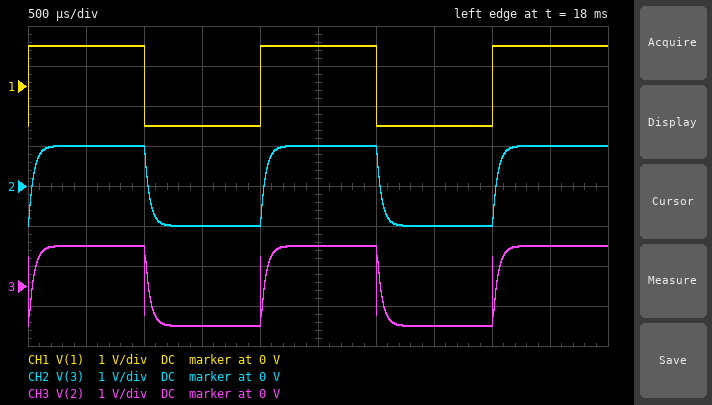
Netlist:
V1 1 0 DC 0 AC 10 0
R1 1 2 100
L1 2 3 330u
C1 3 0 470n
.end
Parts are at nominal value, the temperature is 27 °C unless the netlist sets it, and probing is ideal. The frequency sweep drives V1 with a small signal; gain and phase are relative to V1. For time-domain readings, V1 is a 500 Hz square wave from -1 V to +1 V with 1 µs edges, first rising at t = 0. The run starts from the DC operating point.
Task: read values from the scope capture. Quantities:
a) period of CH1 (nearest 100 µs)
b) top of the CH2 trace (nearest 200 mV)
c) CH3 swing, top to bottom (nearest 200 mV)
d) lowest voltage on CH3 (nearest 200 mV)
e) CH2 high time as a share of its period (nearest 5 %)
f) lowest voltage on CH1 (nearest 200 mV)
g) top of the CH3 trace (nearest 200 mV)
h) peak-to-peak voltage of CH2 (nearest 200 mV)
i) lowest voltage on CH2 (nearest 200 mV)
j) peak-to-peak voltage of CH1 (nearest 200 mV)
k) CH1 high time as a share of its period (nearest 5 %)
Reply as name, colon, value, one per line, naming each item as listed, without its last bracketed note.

period of CH1: 2.0 ms
top of the CH2 trace: 1.0 V
CH3 swing, top to bottom: 2.0 V
lowest voltage on CH3: -1.0 V
CH2 high time as a share of its period: 50 %
lowest voltage on CH1: -1.0 V
top of the CH3 trace: 1.0 V
peak-to-peak voltage of CH2: 2.0 V
lowest voltage on CH2: -1.0 V
peak-to-peak voltage of CH1: 2.0 V
CH1 high time as a share of its period: 50 %
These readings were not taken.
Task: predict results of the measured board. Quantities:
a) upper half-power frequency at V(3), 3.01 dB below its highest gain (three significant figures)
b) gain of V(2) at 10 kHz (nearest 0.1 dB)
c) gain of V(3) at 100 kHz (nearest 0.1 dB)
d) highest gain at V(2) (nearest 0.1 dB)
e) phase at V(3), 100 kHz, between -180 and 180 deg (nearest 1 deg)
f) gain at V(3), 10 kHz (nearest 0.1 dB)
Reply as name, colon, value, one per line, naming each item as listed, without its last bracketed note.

upper half-power frequency at V(3), 3.01 dB below its highest gain: 3.64 kHz
gain of V(2) at 10 kHz: -17.7 dB
gain of V(3) at 100 kHz: -36.5 dB
highest gain at V(2): 0 dB
phase at V(3), 100 kHz, between -180 and 180 deg: -154 deg
gain at V(3), 10 kHz: -9.5 dB
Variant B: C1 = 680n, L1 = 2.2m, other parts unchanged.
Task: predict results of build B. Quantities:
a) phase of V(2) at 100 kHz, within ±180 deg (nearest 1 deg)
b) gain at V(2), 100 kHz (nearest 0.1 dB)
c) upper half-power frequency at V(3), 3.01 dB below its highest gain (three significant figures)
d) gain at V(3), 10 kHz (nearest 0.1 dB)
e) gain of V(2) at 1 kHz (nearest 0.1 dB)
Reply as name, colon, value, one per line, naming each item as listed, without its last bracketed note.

phase of V(2) at 100 kHz, within ±180 deg: 4 deg
gain at V(2), 100 kHz: 0 dB
upper half-power frequency at V(3), 3.01 dB below its highest gain: 3.17 kHz
gain at V(3), 10 kHz: -16.3 dB
gain of V(2) at 1 kHz: -0.8 dB
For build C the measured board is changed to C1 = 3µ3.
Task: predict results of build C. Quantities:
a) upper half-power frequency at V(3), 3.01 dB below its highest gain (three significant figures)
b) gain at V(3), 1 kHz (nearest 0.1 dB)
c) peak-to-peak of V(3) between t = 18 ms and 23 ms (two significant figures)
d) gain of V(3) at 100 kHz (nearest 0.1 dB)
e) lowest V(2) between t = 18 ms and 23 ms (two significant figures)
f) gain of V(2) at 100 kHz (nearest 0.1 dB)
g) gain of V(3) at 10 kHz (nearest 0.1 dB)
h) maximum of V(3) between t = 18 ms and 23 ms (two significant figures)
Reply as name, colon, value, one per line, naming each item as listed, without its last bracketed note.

upper half-power frequency at V(3), 3.01 dB below its highest gain: 487 Hz
gain at V(3), 1 kHz: -7.2 dB
peak-to-peak of V(3) between t = 18 ms and 23 ms: 1.8 V
gain of V(3) at 100 kHz: -53.6 dB
lowest V(2) between t = 18 ms and 23 ms: -910 mV
gain of V(2) at 100 kHz: -0.9 dB
gain of V(3) at 10 kHz: -26.4 dB
maximum of V(3) between t = 18 ms and 23 ms: 910 mV
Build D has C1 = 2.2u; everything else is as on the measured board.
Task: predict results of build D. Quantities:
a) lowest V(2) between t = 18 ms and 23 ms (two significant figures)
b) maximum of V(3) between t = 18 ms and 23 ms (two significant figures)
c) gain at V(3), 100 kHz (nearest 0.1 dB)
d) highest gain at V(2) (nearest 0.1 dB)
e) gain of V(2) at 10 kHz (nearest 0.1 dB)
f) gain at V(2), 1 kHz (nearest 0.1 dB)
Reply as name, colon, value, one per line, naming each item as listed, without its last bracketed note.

lowest V(2) between t = 18 ms and 23 ms: -980 mV
maximum of V(3) between t = 18 ms and 23 ms: 980 mV
gain at V(3), 100 kHz: -50.0 dB
highest gain at V(2): 0 dB
gain of V(2) at 10 kHz: -17.5 dB
gain at V(2), 1 kHz: -4.8 dB
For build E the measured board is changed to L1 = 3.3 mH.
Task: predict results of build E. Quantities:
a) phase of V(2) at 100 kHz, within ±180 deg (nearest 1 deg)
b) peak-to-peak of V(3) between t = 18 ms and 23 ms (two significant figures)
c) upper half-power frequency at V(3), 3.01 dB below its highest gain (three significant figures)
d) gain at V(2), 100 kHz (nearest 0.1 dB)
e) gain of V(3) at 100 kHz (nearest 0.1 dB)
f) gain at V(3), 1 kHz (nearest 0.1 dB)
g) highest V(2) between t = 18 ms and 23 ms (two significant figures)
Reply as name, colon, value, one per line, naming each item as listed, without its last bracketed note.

phase of V(2) at 100 kHz, within ±180 deg: 3 deg
peak-to-peak of V(3) between t = 18 ms and 23 ms: 2.4 V
upper half-power frequency at V(3), 3.01 dB below its highest gain: 4.51 kHz
gain at V(2), 100 kHz: 0 dB
gain of V(3) at 100 kHz: -55.7 dB
gain at V(3), 1 kHz: 0.1 dB
highest V(2) between t = 18 ms and 23 ms: 1.1 V
